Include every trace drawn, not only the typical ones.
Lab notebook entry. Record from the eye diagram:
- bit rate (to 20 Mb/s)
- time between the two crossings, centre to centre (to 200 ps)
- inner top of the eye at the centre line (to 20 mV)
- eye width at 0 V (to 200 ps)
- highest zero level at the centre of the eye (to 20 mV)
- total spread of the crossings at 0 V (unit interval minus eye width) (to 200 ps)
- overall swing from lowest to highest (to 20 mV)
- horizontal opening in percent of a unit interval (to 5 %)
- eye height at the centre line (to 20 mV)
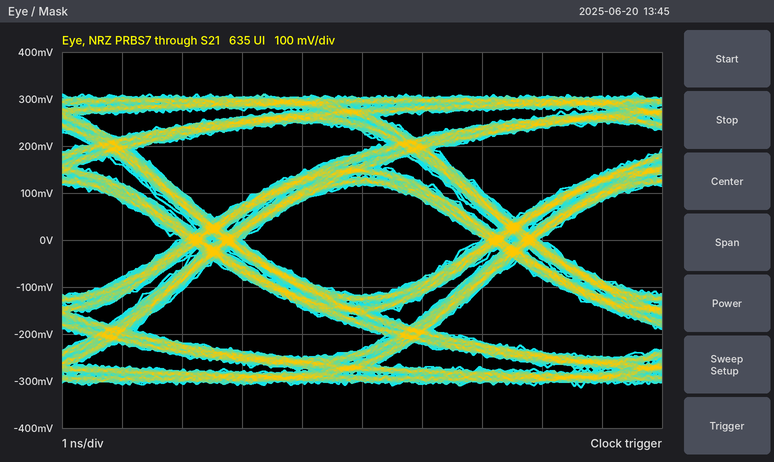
200 Mb/s
5.0 ns
120 mV
4.0 ns
-120 mV
1.0 ns
620 mV
80 %
240 mV
